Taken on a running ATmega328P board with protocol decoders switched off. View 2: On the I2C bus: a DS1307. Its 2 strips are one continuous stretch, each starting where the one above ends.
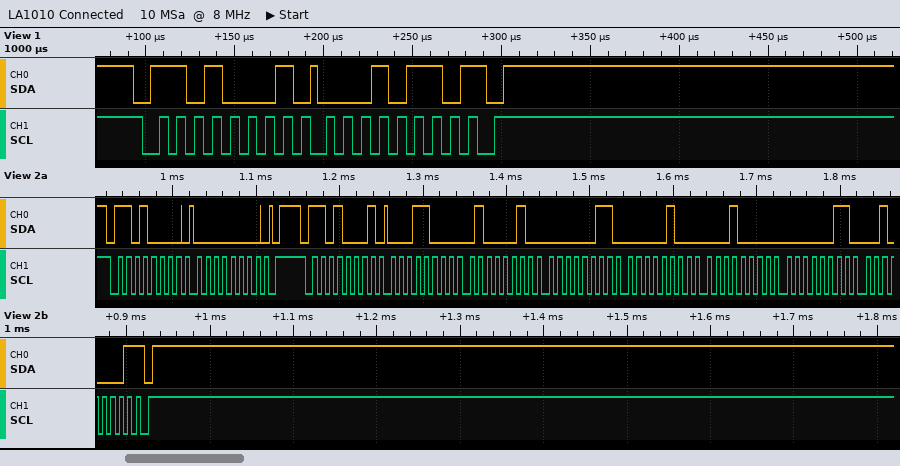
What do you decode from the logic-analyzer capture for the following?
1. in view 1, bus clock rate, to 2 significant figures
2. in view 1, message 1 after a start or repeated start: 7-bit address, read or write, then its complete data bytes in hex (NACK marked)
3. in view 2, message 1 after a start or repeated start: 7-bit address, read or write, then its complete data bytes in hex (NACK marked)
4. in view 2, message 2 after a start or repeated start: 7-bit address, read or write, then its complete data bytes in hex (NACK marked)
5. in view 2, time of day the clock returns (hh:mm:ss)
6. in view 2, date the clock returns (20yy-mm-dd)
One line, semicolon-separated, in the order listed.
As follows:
100 kHz; 0x68 read: 16 NACK; 0x68 write: 00; 0x68 read: 18 42 03 04 10 03 21 NACK; 03:42:18; 2021-03-10
